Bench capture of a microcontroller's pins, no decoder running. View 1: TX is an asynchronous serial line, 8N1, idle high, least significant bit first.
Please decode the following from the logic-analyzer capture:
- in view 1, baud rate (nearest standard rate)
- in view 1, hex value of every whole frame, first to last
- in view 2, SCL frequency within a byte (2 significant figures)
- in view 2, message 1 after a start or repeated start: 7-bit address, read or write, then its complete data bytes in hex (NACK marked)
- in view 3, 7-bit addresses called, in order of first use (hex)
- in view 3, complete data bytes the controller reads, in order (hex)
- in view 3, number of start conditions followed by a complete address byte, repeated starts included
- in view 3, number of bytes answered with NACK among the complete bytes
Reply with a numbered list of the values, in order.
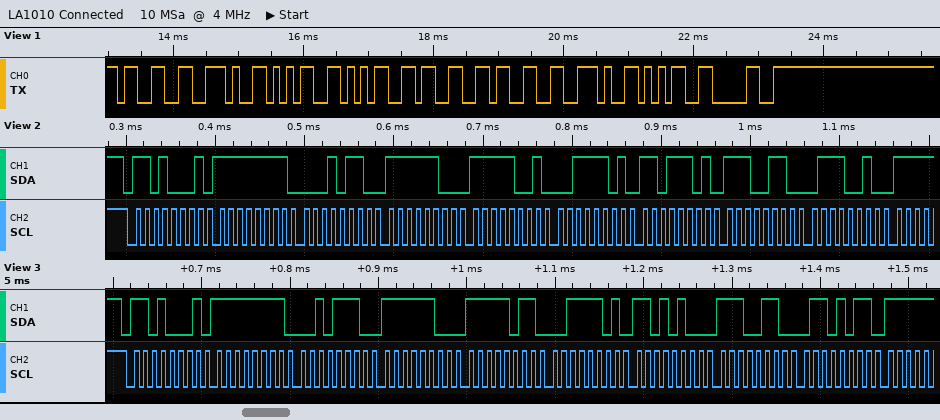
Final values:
1. 9600 baud
2. 33 2E 35 35 33 33 2E 35 30
3. 100 kHz
4. 0x68 read: FF 16 FC F9 3D DD E6 72
5. 0x68
6. FF 2E FC FB 3D D4 E6 6B
7. 1
8. 0
